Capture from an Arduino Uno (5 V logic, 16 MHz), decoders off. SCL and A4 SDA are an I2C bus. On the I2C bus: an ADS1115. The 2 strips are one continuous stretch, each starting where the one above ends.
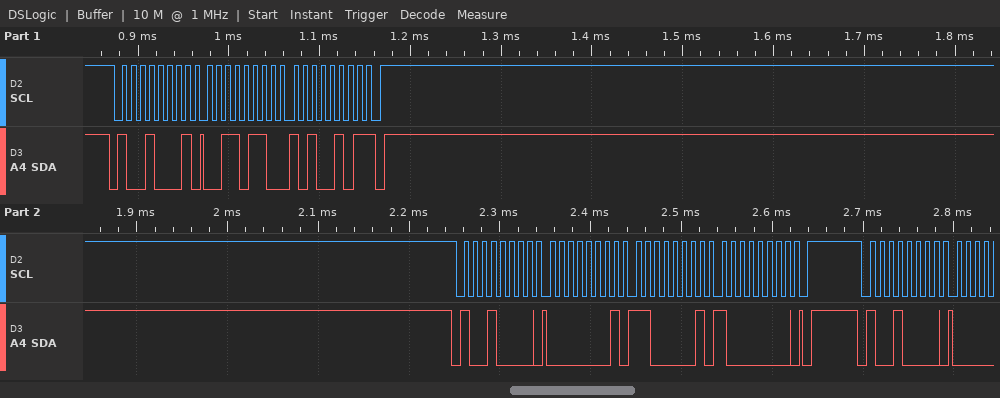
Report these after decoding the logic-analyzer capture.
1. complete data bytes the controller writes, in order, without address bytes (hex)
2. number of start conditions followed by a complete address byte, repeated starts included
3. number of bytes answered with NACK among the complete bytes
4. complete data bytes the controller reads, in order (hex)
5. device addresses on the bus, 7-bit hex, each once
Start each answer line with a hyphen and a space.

- 01 C1 80
- 3
- 1
- 36 A5
- 0x48
